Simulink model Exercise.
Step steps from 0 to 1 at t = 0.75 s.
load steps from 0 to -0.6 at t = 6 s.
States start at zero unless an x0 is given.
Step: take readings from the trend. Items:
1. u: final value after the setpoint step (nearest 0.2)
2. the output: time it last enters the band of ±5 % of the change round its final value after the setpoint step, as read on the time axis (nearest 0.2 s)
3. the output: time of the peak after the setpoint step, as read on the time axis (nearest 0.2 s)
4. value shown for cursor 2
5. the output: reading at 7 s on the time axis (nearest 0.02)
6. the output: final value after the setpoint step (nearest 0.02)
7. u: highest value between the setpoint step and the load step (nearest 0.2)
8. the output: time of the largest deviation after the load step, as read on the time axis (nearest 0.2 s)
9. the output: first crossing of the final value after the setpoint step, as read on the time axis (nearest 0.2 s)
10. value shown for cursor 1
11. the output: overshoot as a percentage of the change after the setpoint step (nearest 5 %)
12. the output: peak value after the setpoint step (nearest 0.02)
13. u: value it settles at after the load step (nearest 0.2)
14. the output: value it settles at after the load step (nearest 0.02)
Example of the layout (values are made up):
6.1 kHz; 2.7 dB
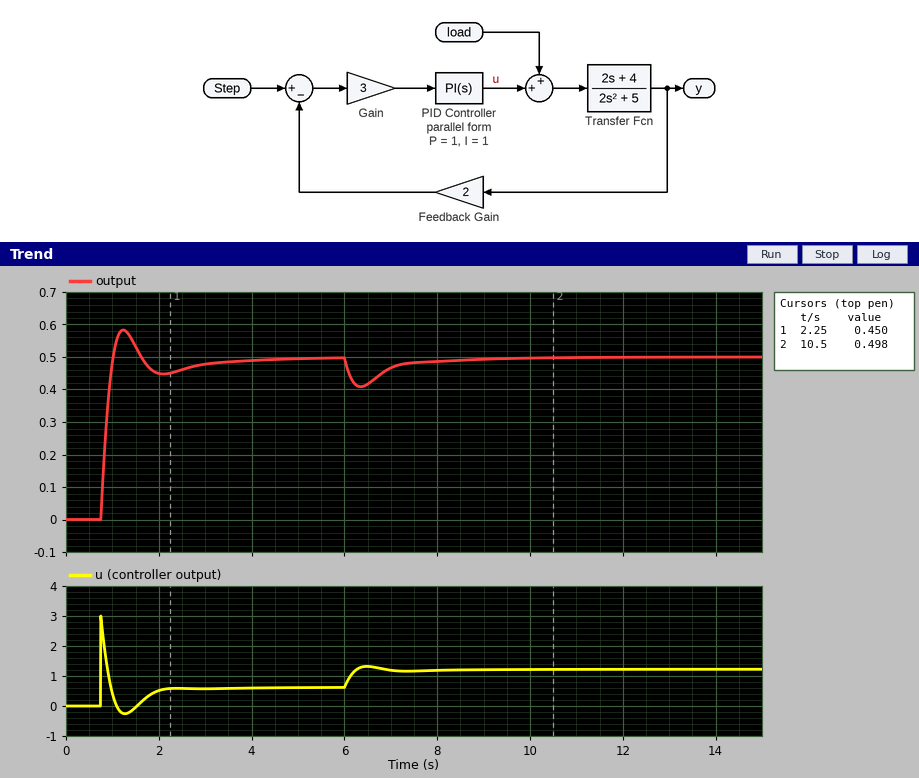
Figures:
0.6; 2.8 s; 1.2 s; 0.498; 0.46; 0.50; 3.0; 6.4 s; 1.0 s; 0.450; 15 %; 0.58; 1.2; 0.50
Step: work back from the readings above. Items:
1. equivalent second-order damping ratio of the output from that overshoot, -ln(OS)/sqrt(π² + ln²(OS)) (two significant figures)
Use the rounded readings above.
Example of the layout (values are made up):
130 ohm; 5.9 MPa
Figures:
0.52
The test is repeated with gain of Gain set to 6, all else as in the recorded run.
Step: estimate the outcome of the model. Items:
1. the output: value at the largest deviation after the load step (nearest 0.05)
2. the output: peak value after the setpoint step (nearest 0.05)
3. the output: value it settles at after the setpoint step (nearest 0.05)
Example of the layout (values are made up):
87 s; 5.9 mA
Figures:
0.45; 0.55; 0.50
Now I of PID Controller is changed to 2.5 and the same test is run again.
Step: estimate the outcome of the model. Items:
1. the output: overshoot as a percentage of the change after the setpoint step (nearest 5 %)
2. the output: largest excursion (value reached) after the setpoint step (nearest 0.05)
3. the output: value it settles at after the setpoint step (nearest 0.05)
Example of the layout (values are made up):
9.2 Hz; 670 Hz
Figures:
25 %; 0.65; 0.50
